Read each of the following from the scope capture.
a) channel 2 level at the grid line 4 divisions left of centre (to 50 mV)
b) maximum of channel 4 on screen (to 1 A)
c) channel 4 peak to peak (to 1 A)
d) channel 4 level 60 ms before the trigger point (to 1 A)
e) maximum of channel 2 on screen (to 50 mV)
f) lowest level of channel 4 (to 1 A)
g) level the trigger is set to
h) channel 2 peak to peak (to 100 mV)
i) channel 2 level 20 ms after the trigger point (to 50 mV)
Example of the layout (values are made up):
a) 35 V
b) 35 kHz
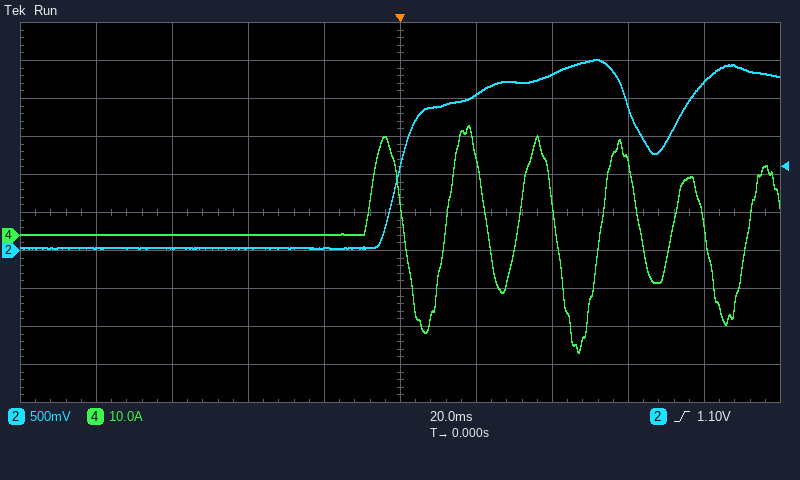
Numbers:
a) 50 mV
b) 29 A
c) 60 A
d) 0 A
e) 2.50 V
f) -31 A
g) 1.10 V
h) 2.50 V
i) 2.05 V
